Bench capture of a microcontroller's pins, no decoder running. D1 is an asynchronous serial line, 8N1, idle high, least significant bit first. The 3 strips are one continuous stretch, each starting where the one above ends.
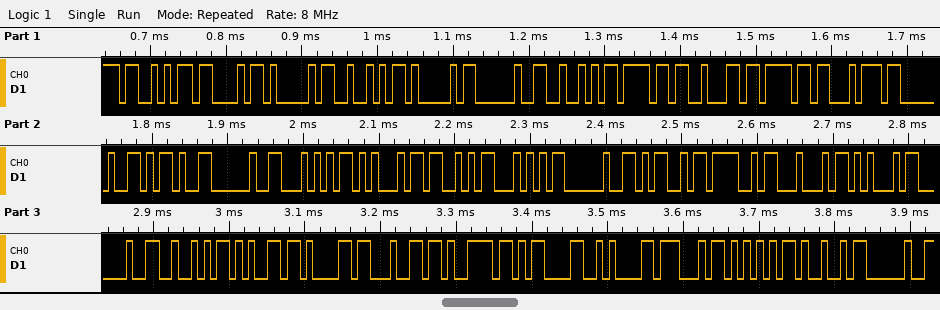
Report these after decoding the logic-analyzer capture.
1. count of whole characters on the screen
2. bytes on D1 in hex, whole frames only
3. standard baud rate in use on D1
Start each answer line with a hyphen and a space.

- 35
- 53 43 41 52 41 20 52 6F 62 6F 74 20 2D 20 54 45 53 54 20 4D 4F 44 45 20 52 65 61 64 79 0D 0A 47 55 49 20
- 115200 baud
